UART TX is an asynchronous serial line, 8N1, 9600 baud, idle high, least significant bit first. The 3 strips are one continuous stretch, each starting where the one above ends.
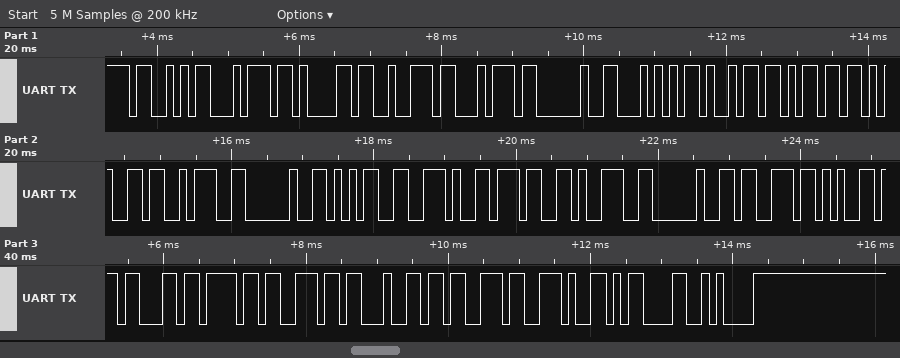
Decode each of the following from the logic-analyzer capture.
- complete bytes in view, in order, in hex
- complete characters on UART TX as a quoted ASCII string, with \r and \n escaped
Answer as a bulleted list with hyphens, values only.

- 53 74 61 72 74 20 54 69 6D 65 3A 20 35 2E 37 39 20 73 65 63 6F 6E 64 73 2E 0D 0A
- "Start Time: 5.79 seconds.\r\n"
